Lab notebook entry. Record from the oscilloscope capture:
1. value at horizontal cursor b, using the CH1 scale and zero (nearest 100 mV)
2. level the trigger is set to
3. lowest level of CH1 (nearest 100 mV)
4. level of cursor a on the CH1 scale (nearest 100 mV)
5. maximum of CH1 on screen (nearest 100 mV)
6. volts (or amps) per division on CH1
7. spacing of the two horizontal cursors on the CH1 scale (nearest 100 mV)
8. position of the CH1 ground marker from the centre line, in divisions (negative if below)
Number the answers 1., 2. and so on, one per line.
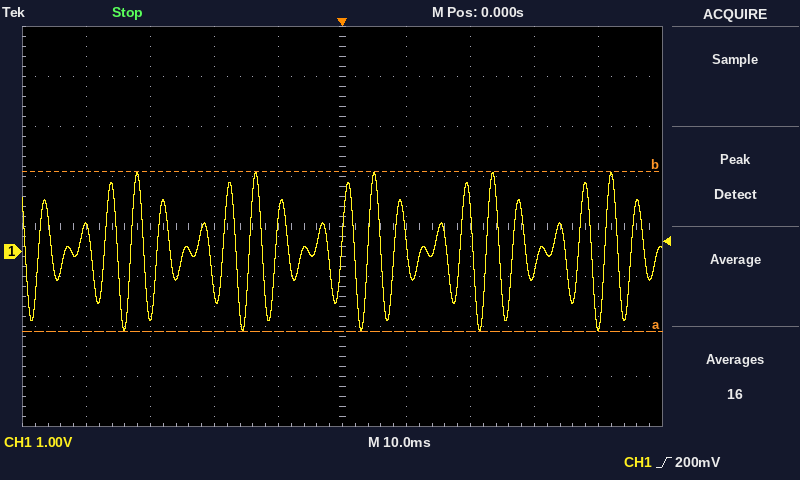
1. 1.6 V
2. 200 mV
3. -1.6 V
4. -1.6 V
5. 1.6 V
6. 1 V
7. 3.2 V
8. -0.5 div
